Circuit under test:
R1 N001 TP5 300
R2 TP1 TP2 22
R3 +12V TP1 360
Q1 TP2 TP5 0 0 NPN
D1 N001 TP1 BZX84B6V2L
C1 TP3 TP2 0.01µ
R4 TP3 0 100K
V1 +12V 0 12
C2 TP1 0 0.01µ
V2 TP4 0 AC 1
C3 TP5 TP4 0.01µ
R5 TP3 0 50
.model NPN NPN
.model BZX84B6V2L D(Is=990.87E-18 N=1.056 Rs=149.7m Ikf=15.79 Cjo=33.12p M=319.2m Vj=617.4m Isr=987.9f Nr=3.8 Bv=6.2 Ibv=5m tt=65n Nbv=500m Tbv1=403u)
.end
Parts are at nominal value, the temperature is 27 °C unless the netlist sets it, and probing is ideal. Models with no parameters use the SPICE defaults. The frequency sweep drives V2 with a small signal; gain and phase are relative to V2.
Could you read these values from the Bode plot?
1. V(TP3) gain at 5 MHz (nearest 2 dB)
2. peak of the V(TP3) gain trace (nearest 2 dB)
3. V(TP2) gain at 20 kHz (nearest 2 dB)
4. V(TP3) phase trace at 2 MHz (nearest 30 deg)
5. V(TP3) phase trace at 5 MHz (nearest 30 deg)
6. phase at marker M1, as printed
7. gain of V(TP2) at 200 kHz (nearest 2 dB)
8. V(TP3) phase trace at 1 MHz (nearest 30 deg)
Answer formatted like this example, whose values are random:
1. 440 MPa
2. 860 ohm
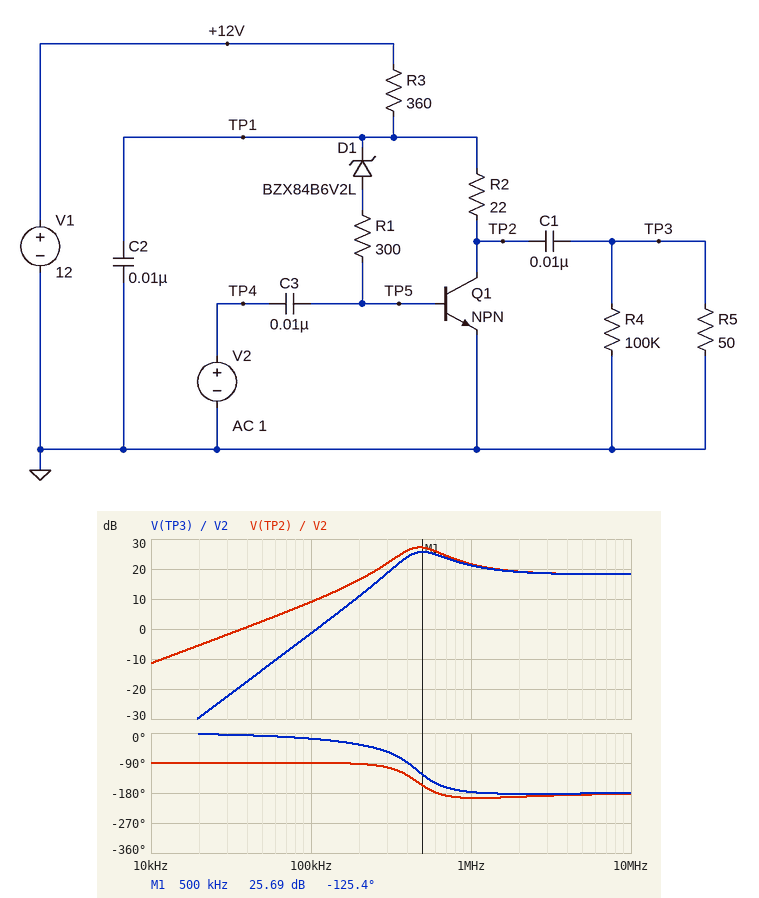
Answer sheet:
1. 18 dB
2. 26 dB
3. -6 dB
4. -180 deg
5. -180 deg
6. -125.4 deg
7. 16 dB
8. -180 deg
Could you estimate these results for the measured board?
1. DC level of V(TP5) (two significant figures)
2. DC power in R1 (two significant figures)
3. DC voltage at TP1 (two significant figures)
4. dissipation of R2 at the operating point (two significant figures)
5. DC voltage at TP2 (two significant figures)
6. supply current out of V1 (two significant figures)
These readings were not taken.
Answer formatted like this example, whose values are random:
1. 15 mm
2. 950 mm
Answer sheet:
1. 840 mV
2. 5.6 µW
3. 7.0 V
4. 4.1 mW
5. 6.7 V
6. 14 mA
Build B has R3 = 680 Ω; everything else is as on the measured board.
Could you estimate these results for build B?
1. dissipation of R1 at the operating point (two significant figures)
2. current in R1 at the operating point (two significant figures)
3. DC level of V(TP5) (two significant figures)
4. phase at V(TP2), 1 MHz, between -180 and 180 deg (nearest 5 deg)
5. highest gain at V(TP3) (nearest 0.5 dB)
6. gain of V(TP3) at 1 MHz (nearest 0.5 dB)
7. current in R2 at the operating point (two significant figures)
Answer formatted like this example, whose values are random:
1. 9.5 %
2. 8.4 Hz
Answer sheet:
1. 1.6 µW
2. 73 µA
3. 830 mV
4. 160 deg
5. 21.0 dB
6. 14.5 dB
7. 7.3 mA
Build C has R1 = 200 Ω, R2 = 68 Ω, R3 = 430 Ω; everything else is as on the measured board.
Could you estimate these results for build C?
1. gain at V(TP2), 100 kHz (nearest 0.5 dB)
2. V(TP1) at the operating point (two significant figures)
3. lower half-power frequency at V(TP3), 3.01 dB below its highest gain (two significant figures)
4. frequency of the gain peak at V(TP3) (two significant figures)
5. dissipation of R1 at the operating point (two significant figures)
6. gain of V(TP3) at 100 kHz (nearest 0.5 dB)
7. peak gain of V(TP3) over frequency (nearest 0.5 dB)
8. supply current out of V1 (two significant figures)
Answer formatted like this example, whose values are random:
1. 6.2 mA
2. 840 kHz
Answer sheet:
1. 9.5 dB
2. 7.0 V
3. 340 kHz
4. 410 kHz
5. 2.6 µW
6. -1.0 dB
7. 29.0 dB
8. 12 mA
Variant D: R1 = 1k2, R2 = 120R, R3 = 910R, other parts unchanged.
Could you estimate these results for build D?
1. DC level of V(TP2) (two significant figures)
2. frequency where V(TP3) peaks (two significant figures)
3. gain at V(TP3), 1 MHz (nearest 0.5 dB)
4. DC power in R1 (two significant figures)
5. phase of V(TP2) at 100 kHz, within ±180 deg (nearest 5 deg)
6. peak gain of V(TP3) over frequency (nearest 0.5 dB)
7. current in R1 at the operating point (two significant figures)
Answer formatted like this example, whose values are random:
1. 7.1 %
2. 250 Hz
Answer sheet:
1. 6.4 V
2. 130 kHz
3. 17.5 dB
4. 3.5 µW
5. -95 deg
6. 27.0 dB
7. 54 µA
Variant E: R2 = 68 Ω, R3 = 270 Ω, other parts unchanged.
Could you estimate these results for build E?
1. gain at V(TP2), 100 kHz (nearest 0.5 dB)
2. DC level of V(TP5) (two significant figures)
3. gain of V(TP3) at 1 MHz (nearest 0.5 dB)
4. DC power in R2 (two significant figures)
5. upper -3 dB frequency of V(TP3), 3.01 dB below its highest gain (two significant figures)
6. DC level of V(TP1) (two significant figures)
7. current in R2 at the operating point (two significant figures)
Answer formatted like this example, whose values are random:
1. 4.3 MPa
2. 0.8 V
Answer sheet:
1. 11.0 dB
2. 850 mV
3. 28.0 dB
4. 22 mW
5. 700 kHz
6. 7.1 V
7. 18 mA
